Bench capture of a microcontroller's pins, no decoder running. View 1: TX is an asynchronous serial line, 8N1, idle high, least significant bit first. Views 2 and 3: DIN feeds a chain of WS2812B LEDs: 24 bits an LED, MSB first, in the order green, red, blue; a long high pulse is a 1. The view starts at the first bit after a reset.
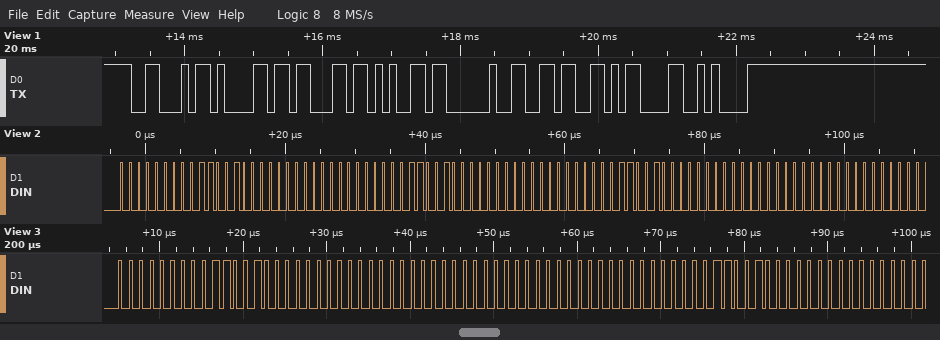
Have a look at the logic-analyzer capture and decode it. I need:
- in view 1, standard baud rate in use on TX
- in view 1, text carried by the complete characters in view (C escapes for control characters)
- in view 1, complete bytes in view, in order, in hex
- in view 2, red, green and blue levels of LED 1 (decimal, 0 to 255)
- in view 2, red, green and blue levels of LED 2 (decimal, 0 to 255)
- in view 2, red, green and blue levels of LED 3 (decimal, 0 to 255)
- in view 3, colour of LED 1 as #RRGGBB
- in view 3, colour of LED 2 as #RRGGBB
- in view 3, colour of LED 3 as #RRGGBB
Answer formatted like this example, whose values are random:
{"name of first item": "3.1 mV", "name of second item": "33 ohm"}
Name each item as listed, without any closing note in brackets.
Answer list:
{"in view 1, standard baud rate in use on TX": "9600 baud", "in view 1, text carried by the complete characters in view": "\"Face 6\\r\\n\"", "in view 1, complete bytes in view, in order, in hex": "46 61 63 65 20 36 0D 0A", "in view 2, red, green and blue levels of LED 1": "100, 0, 0", "in view 2, red, green and blue levels of LED 2": "100, 0, 0", "in view 2, red, green and blue levels of LED 3": "100, 0, 0", "in view 3, colour of LED 1 as #RRGGBB": "#640000", "in view 3, colour of LED 2 as #RRGGBB": "#000000", "in view 3, colour of LED 3 as #RRGGBB": "#640000"}
